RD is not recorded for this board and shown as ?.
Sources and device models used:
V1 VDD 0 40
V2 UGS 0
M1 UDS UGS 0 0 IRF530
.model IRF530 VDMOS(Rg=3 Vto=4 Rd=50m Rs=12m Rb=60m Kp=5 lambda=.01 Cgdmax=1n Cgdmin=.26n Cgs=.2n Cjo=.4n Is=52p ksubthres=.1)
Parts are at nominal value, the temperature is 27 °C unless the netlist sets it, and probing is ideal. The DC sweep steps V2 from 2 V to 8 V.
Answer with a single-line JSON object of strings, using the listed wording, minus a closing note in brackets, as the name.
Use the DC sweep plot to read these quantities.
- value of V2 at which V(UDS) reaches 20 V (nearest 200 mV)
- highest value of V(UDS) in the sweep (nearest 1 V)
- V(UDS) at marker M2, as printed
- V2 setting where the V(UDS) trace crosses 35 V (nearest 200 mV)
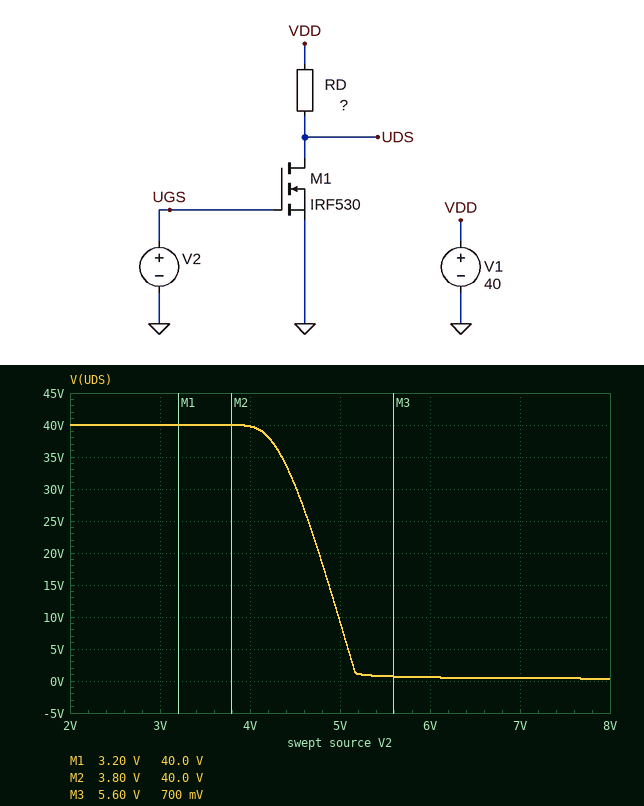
{"value of V2 at which V(UDS) reaches 20 V": "4.8 V", "highest value of V(UDS) in the sweep": "40 V", "V(UDS) at marker M2, as printed": "40.0 V", "V2 setting where the V(UDS) trace crosses 35 V": "4.4 V"}
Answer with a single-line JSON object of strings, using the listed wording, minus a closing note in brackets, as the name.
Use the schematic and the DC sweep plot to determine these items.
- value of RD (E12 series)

{"value of RD": "12 Ω"}
